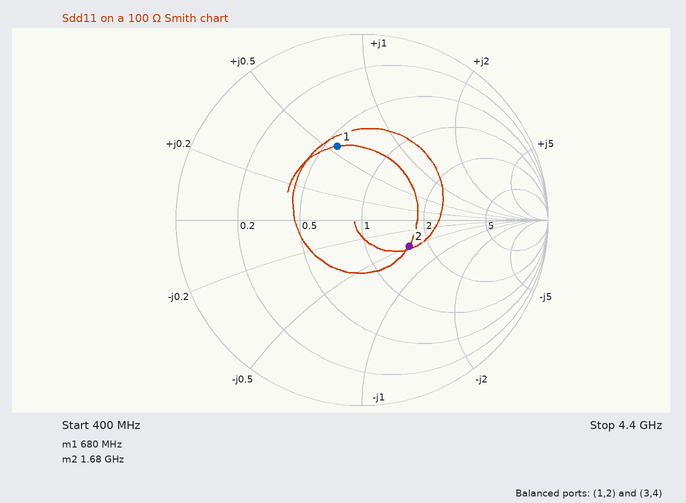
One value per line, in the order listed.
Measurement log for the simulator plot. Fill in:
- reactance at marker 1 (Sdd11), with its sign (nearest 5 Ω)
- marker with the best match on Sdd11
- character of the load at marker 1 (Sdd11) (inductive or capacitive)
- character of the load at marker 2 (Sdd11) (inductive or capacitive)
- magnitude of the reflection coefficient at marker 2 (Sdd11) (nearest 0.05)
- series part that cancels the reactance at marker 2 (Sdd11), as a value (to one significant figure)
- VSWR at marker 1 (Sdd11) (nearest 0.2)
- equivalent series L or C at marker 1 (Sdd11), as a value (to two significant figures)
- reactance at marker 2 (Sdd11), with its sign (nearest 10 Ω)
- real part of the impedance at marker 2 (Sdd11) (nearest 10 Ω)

+55 Ω
marker 2
inductive
capacitive
0.30
5 nH
2.4
13 nH
-50 Ω
160 Ω
